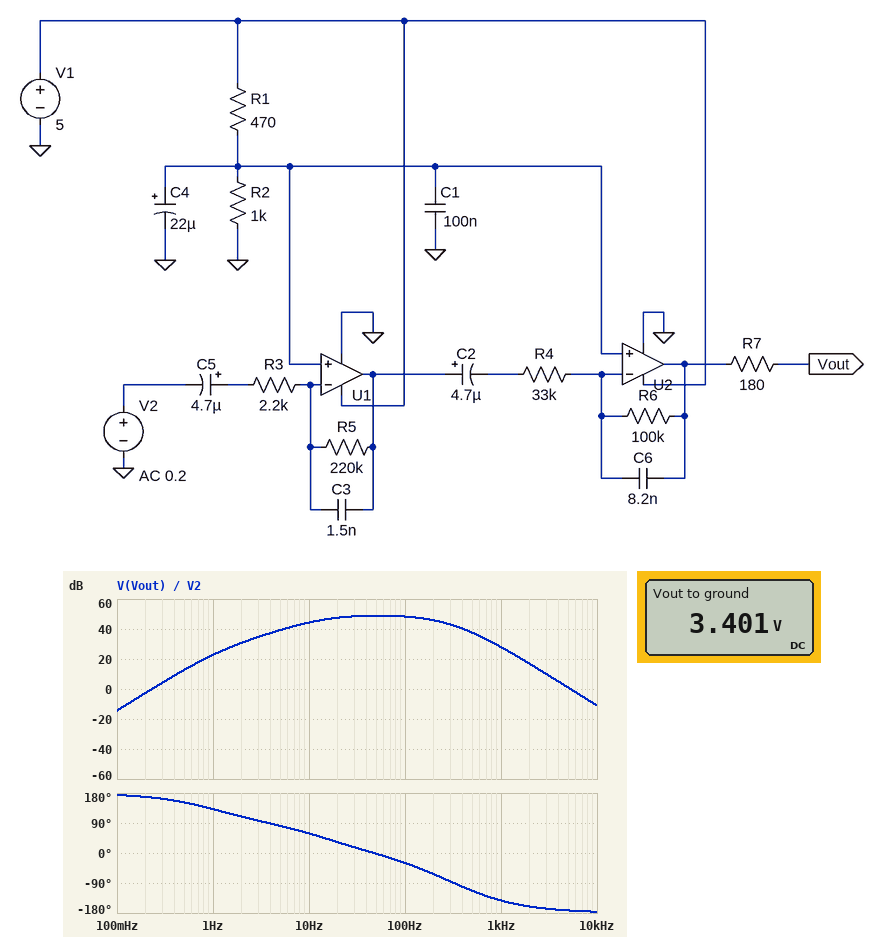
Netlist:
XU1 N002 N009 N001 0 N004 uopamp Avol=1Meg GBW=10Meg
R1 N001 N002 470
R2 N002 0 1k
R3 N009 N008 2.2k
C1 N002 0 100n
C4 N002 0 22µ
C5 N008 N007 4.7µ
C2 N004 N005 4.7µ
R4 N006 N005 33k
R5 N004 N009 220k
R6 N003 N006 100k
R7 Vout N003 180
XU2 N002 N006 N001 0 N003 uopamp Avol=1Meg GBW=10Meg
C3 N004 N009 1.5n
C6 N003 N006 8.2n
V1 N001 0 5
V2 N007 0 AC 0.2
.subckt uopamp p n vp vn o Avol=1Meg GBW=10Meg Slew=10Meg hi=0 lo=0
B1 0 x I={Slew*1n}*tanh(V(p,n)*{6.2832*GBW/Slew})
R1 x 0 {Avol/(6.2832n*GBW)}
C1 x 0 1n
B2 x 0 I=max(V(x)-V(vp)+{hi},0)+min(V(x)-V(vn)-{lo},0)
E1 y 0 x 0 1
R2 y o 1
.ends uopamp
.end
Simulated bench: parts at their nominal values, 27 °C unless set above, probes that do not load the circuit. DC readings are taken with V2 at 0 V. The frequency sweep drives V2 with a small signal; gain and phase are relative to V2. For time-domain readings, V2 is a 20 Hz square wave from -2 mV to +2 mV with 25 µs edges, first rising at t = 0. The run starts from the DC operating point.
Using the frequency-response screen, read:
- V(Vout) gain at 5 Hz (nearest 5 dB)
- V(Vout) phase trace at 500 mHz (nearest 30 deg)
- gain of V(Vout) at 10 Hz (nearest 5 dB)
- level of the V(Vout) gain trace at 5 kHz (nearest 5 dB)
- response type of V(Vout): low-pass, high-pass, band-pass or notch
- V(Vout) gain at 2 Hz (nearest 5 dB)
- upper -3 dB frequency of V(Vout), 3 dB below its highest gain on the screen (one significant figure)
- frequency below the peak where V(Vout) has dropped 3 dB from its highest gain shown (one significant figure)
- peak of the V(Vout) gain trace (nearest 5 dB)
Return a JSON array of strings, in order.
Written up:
["40 dB", "150 deg", "45 dB", "0 dB", "band-pass", "30 dB", "200 Hz", "10 Hz", "50 dB"]
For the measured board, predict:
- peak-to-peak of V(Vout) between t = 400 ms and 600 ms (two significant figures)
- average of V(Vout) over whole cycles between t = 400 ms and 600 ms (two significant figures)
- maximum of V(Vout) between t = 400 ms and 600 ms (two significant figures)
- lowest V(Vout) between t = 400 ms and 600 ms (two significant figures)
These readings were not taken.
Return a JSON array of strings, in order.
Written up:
["1.8 V", "3.4 V", "4.3 V", "2.5 V"]
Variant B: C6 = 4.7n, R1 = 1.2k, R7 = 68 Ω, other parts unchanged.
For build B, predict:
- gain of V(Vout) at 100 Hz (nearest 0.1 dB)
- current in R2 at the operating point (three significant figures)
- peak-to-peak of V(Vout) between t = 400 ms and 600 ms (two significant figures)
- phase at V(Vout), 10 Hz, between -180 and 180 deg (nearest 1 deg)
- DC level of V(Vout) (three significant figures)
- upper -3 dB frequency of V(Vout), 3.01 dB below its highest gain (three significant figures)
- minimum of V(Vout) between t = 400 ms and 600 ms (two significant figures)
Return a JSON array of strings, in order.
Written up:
["49.0 dB", "2.27 mA", "1.9 V", "60 deg", "2.27 V", "277 Hz", "1.3 V"]
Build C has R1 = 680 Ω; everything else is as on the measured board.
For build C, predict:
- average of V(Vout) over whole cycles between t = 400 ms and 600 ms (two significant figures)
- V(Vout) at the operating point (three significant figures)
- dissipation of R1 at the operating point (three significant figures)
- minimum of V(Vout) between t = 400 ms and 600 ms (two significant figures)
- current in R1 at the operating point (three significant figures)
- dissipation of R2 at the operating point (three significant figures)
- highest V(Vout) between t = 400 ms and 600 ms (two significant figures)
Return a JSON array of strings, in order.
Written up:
["3.0 V", "2.98 V", "6.02 mW", "2.1 V", "2.98 mA", "8.86 mW", "3.9 V"]
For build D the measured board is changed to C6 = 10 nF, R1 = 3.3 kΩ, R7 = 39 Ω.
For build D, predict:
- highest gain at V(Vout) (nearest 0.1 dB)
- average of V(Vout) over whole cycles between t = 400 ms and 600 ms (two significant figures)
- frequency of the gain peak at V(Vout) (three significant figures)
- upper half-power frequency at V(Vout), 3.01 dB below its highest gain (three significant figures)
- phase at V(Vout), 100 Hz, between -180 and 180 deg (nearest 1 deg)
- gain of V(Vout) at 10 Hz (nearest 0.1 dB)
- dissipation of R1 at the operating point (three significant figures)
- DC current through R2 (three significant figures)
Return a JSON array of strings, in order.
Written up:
["48.8 dB", "1.2 V", "48.1 Hz", "170 Hz", "-35 deg", "44.3 dB", "4.46 mW", "1.16 mA"]
